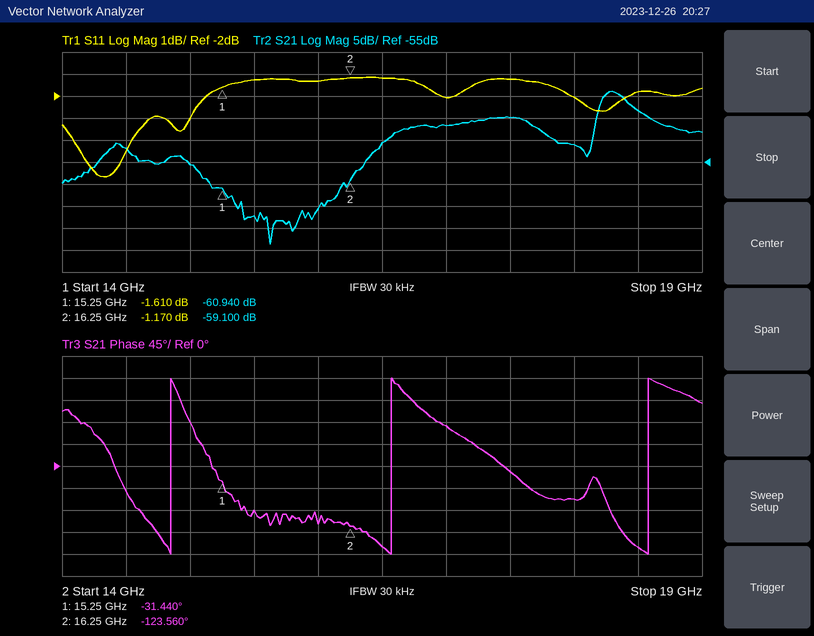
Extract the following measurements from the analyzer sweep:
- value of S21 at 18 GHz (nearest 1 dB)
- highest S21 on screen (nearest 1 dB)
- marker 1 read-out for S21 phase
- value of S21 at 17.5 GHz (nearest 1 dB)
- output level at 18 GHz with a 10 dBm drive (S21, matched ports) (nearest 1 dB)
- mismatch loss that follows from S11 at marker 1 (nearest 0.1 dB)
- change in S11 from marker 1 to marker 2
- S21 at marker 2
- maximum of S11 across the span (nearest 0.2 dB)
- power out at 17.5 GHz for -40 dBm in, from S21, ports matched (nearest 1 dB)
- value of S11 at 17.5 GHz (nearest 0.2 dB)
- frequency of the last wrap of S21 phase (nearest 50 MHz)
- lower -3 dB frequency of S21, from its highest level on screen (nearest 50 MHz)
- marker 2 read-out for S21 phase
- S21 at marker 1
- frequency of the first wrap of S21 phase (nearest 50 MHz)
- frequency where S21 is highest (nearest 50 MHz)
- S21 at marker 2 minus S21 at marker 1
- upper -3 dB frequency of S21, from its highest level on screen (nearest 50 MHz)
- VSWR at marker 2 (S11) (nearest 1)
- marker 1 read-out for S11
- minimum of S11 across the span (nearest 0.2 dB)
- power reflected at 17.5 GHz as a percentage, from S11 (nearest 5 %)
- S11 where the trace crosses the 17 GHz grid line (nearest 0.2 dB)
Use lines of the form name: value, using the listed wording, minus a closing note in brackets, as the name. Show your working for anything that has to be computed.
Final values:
value of S21 at 18 GHz: -51 dB
highest S21 on screen: -39 dB
marker 1 read-out for S21 phase: -31.440°
value of S21 at 17.5 GHz: -45 dB
output level at 18 GHz with a 10 dBm drive (S21, matched ports): 10 dBm + (-51 dB) = -41 dBm
mismatch loss that follows from S11 at marker 1: −10 log10(1 − 10^(-1.61/10)) ≈ 5.1 dB
change in S11 from marker 1 to marker 2: -1.17 − (-1.61) = 0.440 dB
S21 at marker 2: -59.100 dB
maximum of S11 across the span: -1.2 dB
power out at 17.5 GHz for -40 dBm in, from S21, ports matched: -40 dBm + (-45 dB) = -85 dBm
value of S11 at 17.5 GHz: -1.2 dB
frequency of the last wrap of S21 phase: 18.60 GHz
lower -3 dB frequency of S21, from its highest level on screen: 18.20 GHz
marker 2 read-out for S21 phase: -123.560°
S21 at marker 1: -60.940 dB
frequency of the first wrap of S21 phase: 14.85 GHz
frequency where S21 is highest: 18.30 GHz
S21 at marker 2 minus S21 at marker 1: -59.1 − (-60.94) = 1.840 dB
upper -3 dB frequency of S21, from its highest level on screen: 18.45 GHz
VSWR at marker 2 (S11): (1 + 0.8740)/(1 − 0.8740) ≈ 15
marker 1 read-out for S11: -1.610 dB
minimum of S11 across the span: -5.6 dB
power reflected at 17.5 GHz as a percentage, from S11: 10^(-1.2/10) ≈ 75.9 %, so 75 % to the nearest 5 %
S11 where the trace crosses the 17 GHz grid line: -2.0 dB
